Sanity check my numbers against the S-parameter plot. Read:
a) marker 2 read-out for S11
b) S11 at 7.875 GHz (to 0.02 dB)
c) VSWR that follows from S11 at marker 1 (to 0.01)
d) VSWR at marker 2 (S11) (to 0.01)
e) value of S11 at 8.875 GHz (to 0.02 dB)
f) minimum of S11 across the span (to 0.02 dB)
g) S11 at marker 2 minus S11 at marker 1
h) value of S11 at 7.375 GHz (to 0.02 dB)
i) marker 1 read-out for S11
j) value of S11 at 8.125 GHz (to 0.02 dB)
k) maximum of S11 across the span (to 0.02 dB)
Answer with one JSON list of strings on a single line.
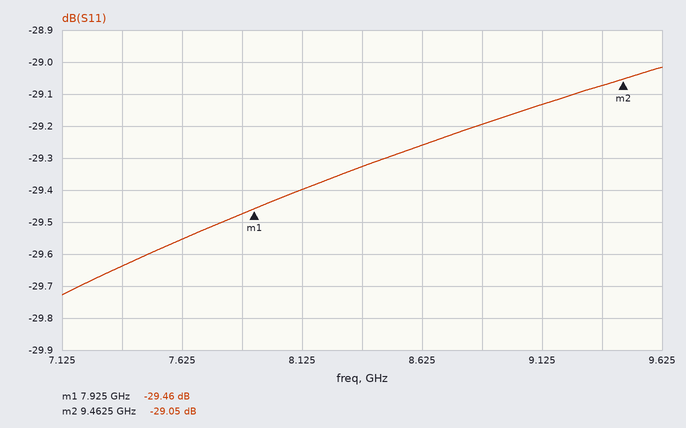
["-29.05 dB", "-29.48 dB", "1.07", "1.07", "-29.20 dB", "-29.72 dB", "0.41 dB", "-29.64 dB", "-29.46 dB", "-29.40 dB", "-29.02 dB"]
